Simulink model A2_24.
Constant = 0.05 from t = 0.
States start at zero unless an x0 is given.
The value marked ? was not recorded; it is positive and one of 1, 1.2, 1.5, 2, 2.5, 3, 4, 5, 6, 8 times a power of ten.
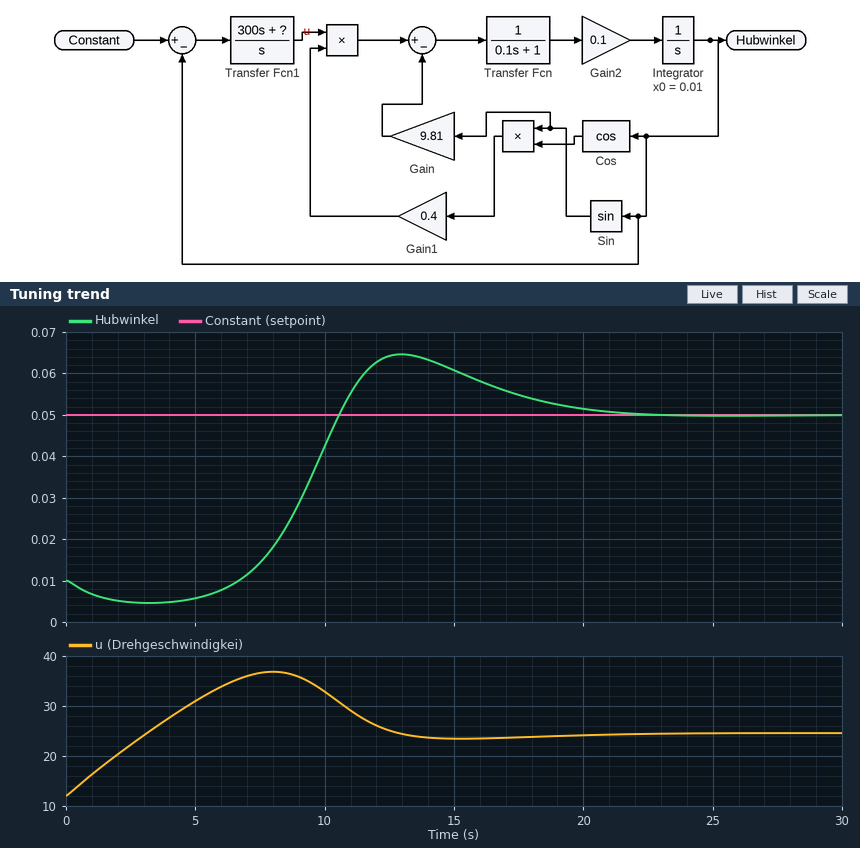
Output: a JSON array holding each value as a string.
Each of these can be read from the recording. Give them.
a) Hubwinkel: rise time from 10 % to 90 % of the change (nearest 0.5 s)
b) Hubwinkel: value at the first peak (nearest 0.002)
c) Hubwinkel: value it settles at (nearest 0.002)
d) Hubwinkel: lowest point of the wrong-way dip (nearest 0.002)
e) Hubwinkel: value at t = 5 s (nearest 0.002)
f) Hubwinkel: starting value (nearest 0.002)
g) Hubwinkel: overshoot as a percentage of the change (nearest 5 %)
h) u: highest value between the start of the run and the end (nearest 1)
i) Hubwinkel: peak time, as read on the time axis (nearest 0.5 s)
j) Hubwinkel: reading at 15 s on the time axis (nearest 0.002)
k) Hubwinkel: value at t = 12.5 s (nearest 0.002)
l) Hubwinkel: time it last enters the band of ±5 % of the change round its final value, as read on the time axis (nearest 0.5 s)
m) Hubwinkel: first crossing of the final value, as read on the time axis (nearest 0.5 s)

["3.0 s", "0.064", "0.050", "0.004", "0.006", "0.010", "35 %", "37", "13.0 s", "0.060", "0.064", "19.5 s", "10.5 s"]
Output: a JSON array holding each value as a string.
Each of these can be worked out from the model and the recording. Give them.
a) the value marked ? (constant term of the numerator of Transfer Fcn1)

["80"]
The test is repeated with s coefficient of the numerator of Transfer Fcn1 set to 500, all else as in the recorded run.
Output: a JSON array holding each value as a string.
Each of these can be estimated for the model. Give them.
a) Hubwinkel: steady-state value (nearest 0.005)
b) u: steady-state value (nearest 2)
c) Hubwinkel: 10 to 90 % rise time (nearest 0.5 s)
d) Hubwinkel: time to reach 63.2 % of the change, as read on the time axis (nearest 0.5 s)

["0.050", "24", "7.0 s", "8.0 s"]
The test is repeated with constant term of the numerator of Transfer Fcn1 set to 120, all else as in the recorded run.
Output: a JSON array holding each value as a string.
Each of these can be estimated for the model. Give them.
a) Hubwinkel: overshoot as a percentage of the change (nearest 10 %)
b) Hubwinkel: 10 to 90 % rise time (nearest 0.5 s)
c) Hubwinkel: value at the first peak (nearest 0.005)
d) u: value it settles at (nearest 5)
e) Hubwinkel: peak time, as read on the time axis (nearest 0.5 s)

["50 %", "2.5 s", "0.070", "25", "10.0 s"]
